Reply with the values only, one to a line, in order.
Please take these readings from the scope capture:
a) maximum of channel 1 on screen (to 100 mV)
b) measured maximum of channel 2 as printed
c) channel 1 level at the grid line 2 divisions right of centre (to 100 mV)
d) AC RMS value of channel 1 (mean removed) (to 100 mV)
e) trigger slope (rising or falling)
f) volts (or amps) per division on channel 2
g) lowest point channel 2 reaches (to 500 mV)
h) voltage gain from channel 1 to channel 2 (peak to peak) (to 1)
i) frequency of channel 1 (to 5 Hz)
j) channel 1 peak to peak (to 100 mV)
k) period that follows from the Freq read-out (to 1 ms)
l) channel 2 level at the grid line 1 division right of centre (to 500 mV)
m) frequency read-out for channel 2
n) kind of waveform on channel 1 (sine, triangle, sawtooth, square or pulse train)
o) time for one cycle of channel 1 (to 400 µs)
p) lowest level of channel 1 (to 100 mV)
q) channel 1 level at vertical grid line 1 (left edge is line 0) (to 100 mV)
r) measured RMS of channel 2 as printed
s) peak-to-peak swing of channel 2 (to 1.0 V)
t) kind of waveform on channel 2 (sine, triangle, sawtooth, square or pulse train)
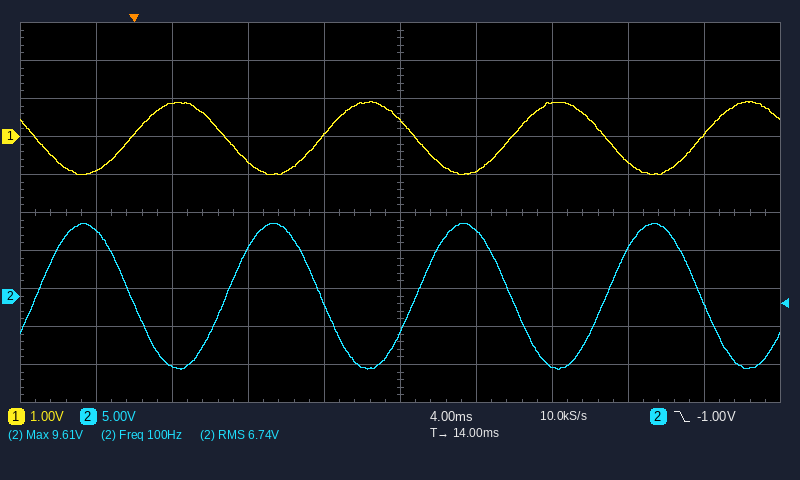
900 mV
9.61 V
900 mV
700 mV
falling
5 V
-9.5 V
10
100 Hz
1.9 V
10 ms
8.5 V
100 Hz
sine
10.0 ms
-1.0 V
-900 mV
6.74 V
19.0 V
sine
